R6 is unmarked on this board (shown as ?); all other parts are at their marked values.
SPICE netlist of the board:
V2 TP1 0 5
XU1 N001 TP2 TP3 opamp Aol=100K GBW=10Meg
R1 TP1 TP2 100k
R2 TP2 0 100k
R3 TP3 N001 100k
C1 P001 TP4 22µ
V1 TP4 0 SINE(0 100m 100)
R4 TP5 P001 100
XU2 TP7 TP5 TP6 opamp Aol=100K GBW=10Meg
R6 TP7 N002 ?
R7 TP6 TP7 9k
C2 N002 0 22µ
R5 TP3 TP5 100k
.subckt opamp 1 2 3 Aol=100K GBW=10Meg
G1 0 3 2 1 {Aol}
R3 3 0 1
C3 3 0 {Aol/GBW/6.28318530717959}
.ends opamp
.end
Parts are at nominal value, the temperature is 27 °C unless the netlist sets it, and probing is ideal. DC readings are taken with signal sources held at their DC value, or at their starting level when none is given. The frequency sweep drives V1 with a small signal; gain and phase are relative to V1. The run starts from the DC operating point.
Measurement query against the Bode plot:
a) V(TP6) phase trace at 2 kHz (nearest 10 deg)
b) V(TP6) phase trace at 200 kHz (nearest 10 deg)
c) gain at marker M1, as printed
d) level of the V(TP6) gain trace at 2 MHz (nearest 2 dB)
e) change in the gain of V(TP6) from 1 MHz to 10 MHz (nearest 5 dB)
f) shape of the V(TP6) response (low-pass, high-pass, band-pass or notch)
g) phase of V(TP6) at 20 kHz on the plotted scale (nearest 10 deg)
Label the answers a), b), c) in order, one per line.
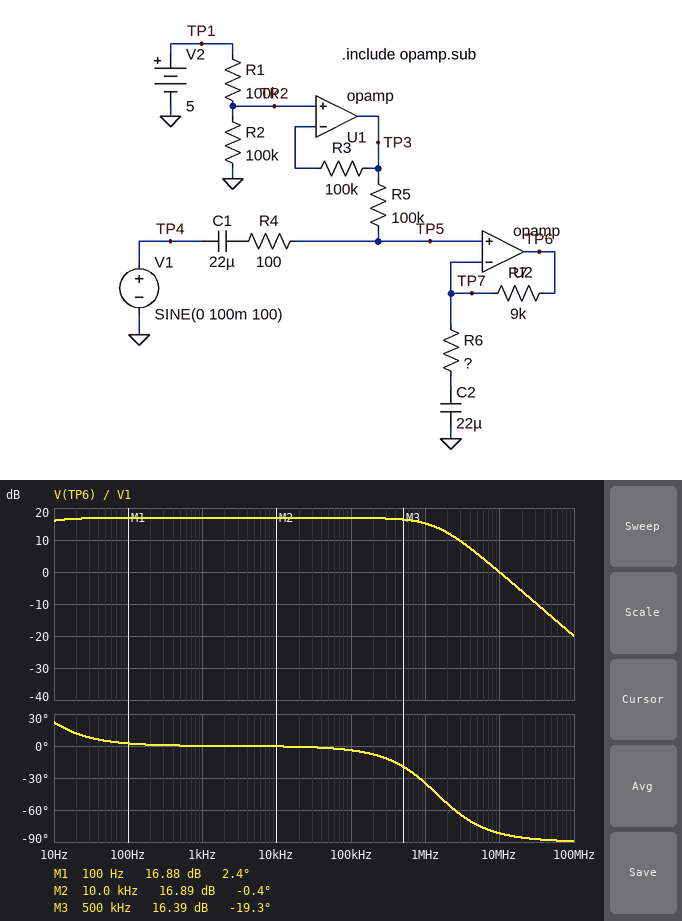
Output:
a) 0 deg
b) -10 deg
c) 16.88 dB
d) 12 dB
e) -15 dB
f) low-pass
g) 0 deg
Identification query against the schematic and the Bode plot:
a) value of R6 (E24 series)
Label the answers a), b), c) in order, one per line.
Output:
a) 1.5 kΩ
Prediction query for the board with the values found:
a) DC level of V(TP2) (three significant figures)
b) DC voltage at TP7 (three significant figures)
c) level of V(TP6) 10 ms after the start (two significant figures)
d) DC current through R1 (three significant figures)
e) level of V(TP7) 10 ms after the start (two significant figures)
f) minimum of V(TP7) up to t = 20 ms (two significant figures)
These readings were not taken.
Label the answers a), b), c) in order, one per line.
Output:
a) 2.50 V
b) 2.50 V
c) 2.5 V
d) 25.0 µA
e) 2.5 V
f) 2.4 V
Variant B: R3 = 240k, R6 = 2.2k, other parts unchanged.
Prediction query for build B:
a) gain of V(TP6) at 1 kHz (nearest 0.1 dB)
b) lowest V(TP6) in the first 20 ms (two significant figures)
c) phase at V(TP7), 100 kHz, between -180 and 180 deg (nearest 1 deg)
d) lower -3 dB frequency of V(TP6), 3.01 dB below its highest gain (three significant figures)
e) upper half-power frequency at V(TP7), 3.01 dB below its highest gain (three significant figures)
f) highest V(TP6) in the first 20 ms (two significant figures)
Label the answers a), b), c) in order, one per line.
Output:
a) 14.1 dB
b) 2.0 V
c) -3 deg
d) 3.16 Hz
e) 1.96 MHz
f) 3.0 V
